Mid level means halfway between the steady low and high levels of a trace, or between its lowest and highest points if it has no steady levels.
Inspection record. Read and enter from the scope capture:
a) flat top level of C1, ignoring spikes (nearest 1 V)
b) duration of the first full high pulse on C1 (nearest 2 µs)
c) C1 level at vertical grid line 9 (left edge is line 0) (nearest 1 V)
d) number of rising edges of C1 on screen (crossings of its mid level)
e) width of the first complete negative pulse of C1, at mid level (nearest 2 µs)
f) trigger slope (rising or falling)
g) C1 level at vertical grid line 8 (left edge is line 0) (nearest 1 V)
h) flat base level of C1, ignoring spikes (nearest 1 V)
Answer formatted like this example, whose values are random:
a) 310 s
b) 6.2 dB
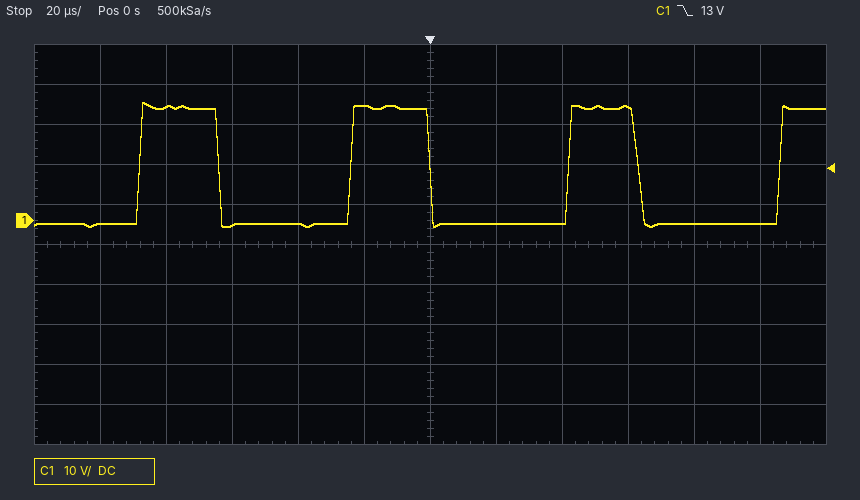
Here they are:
a) 28 V
b) 24 µs
c) 28 V
d) 4
e) 40 µs
f) falling
g) -1 V
h) -1 V
